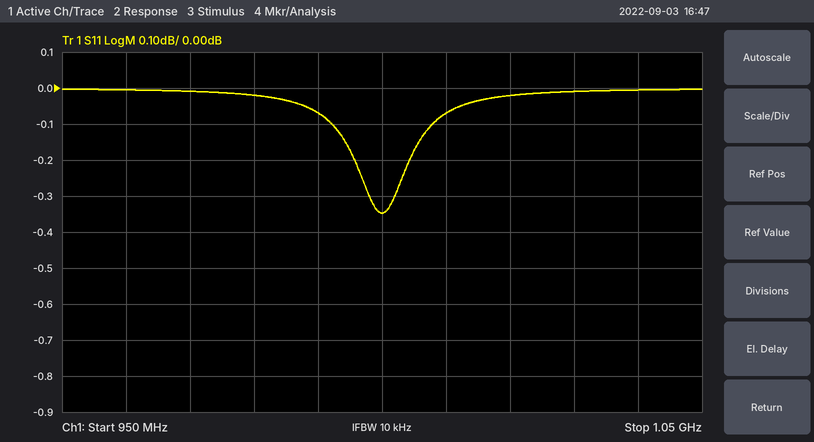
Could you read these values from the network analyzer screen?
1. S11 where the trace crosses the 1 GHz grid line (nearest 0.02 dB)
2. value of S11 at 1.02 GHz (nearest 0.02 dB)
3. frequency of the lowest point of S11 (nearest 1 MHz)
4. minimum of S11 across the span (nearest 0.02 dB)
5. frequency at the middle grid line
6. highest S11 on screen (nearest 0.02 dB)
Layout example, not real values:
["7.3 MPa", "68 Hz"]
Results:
["-0.34 dB", "-0.02 dB", "1.000 GHz", "-0.34 dB", "1 GHz", "0.00 dB"]
